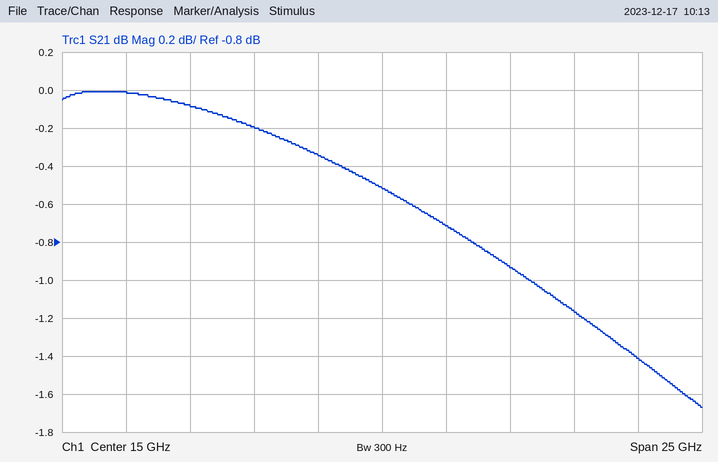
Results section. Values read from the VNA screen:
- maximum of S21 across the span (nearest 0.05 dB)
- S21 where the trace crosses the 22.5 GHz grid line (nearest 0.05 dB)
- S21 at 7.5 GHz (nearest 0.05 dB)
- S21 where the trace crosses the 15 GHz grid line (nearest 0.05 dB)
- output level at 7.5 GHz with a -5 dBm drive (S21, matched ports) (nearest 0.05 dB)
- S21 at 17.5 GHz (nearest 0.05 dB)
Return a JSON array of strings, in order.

["0.00 dB", "-1.15 dB", "-0.10 dB", "-0.50 dB", "-5.10 dBm", "-0.70 dB"]
